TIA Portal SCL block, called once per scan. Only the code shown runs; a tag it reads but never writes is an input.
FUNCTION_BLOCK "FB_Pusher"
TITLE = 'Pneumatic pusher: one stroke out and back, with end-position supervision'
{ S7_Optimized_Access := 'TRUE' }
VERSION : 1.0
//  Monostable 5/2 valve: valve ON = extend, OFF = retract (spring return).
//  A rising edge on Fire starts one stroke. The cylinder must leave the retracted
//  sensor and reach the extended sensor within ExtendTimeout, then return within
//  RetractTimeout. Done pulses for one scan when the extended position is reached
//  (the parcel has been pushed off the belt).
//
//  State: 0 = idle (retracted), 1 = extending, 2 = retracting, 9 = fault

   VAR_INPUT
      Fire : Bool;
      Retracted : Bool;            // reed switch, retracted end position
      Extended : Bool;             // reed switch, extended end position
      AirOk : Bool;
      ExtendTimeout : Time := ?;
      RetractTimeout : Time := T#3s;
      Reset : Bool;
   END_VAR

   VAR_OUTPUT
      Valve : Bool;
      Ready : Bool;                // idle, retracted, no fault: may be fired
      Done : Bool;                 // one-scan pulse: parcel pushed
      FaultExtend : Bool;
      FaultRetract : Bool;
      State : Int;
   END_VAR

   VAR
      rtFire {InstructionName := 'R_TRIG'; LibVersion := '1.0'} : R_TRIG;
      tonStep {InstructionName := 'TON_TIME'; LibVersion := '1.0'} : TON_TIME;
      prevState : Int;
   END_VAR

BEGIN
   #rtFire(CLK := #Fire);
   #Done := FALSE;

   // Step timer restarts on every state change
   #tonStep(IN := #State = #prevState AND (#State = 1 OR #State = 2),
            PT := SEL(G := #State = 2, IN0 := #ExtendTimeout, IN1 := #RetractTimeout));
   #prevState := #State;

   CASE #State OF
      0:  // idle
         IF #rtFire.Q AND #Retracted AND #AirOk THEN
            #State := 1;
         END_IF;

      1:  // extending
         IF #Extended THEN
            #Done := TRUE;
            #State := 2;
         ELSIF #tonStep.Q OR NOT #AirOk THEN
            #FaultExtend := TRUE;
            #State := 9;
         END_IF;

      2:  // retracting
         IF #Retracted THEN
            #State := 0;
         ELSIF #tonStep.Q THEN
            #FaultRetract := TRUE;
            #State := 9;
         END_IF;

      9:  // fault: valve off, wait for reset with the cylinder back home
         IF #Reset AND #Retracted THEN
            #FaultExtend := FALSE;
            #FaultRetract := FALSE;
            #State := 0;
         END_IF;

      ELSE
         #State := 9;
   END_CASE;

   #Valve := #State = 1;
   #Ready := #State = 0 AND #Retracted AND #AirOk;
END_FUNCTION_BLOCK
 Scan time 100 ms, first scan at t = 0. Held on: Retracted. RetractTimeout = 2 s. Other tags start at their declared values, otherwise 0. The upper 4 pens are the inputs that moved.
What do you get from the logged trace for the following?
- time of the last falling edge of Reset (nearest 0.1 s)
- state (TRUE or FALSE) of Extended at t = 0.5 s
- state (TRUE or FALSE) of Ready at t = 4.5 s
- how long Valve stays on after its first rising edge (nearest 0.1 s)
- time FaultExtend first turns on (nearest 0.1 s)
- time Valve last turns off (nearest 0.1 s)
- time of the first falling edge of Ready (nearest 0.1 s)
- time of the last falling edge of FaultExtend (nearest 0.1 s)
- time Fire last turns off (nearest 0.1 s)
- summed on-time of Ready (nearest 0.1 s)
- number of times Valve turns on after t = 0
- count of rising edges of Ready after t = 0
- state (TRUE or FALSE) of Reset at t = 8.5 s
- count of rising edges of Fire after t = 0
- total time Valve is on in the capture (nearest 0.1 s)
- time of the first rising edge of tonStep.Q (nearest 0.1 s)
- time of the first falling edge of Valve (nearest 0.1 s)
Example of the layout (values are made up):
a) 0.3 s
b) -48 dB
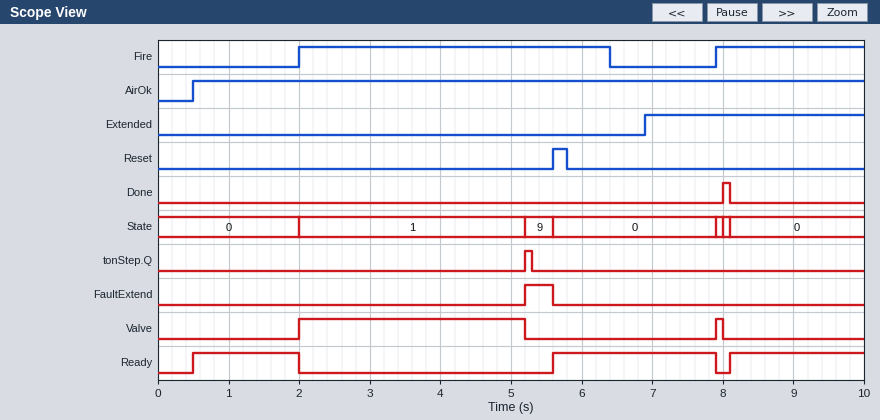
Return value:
a) 5.8 s
b) FALSE
c) FALSE
d) 3.2 s
e) 5.2 s
f) 8.0 s
g) 2.0 s
h) 5.6 s
i) 6.4 s
j) 5.7 s
k) 2
l) 3
m) FALSE
n) 2
o) 3.3 s
p) 5.2 s
q) 5.2 s
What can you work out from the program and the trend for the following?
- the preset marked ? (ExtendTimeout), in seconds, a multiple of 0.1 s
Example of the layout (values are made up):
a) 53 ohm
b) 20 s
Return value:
a) 3.0 s
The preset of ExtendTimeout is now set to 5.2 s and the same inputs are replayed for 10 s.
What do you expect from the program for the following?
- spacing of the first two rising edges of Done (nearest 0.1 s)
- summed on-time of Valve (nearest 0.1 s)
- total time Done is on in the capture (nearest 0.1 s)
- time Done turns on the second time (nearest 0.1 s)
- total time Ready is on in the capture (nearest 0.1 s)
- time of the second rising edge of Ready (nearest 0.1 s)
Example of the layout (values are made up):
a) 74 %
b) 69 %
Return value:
a) 1.1 s
b) 5.0 s
c) 0.2 s
d) 8.0 s
e) 4.3 s
f) 7.0 s
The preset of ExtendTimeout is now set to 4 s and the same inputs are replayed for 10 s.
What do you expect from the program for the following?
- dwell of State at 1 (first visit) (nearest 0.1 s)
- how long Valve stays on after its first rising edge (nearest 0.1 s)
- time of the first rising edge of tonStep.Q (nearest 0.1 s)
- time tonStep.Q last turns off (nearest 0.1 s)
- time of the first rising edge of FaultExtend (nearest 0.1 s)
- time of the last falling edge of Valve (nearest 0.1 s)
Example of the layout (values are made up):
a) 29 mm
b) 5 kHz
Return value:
a) 4.2 s
b) 4.2 s
c) 6.2 s
d) 6.3 s
e) 6.2 s
f) 6.2 s
